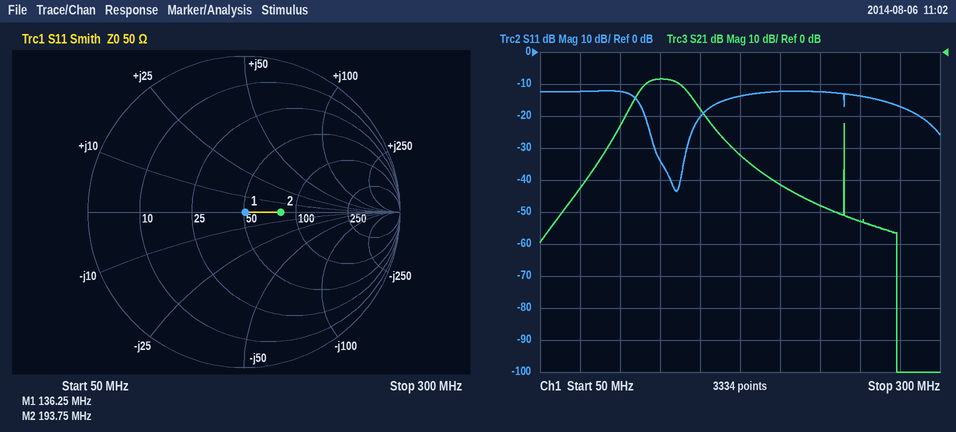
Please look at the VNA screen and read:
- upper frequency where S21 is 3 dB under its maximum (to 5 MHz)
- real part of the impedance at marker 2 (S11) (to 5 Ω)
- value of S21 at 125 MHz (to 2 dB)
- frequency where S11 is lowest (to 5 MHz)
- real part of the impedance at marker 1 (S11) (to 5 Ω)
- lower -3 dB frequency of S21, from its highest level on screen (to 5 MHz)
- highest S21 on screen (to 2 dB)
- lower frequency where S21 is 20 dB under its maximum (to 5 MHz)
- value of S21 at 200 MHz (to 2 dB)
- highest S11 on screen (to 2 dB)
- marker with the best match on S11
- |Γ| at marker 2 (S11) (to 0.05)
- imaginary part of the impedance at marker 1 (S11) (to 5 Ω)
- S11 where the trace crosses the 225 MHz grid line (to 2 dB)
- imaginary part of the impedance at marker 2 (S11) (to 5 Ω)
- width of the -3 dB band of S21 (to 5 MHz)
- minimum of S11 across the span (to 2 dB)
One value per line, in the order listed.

140 MHz
80 Ω
-8 dB
135 MHz
50 Ω
115 MHz
-8 dB
95 MHz
-42 dB
-12 dB
marker 1
0.25
0 Ω
-12 dB
0 Ω
25 MHz
-44 dB
